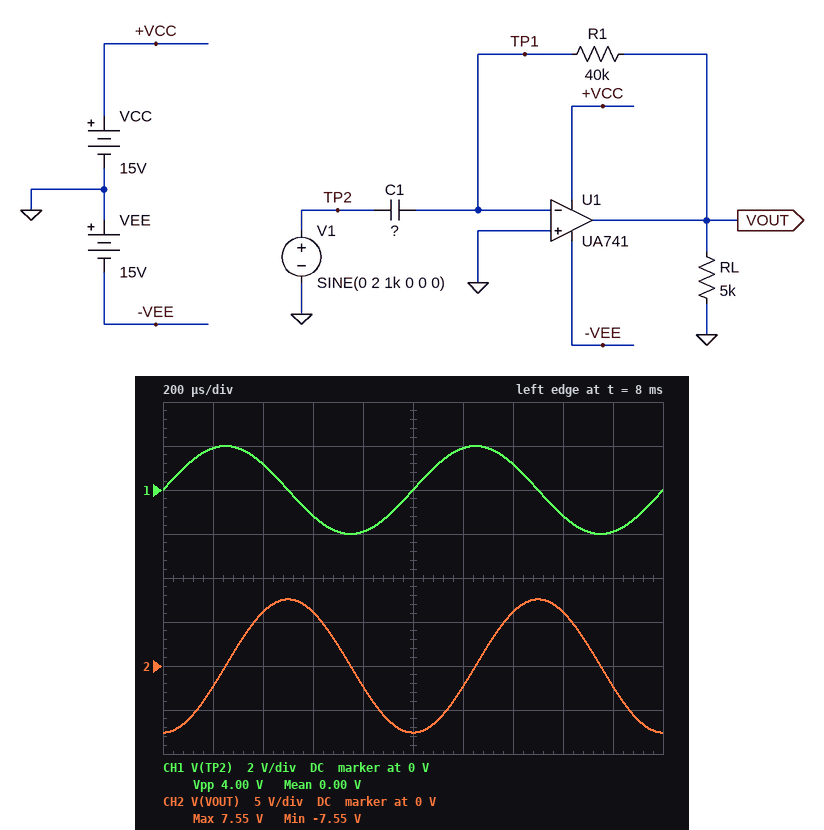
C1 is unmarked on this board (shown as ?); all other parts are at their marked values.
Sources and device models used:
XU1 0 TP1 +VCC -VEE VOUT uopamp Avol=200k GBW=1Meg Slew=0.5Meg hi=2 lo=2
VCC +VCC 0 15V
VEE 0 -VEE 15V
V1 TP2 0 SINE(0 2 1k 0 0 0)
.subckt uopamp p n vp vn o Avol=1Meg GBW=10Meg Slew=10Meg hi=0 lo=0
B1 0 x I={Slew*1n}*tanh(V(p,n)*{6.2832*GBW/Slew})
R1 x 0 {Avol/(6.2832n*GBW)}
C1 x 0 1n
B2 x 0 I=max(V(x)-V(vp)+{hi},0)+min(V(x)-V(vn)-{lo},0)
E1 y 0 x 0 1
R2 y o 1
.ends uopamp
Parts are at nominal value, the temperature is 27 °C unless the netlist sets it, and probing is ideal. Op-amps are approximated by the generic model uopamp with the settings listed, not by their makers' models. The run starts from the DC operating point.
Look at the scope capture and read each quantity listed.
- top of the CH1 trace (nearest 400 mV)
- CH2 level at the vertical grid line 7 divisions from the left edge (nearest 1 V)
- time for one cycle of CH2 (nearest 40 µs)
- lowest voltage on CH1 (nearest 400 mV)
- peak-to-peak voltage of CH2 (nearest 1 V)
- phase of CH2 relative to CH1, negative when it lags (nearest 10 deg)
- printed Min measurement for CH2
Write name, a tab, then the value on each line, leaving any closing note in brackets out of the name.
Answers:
top of the CH1 trace	2.0 V
CH2 level at the vertical grid line 7 divisions from the left edge	6 V
time for one cycle of CH2	1.00 ms
lowest voltage on CH1	-2.0 V
peak-to-peak voltage of CH2	15 V
phase of CH2 relative to CH1, negative when it lags	-90 deg
printed Min measurement for CH2	-7.55 V
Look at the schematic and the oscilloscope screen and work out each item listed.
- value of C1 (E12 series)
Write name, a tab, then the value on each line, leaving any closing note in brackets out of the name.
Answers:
value of C1	15 nF
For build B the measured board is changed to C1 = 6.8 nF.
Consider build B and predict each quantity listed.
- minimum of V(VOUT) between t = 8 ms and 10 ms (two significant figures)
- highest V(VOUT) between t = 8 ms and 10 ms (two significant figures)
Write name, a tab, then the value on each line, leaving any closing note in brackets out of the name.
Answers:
minimum of V(VOUT) between t = 8 ms and 10 ms	-3.4 V
highest V(VOUT) between t = 8 ms and 10 ms	3.4 V
